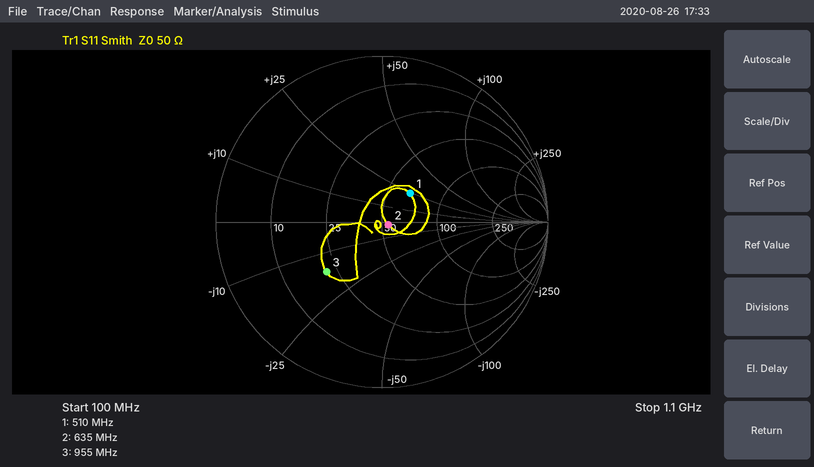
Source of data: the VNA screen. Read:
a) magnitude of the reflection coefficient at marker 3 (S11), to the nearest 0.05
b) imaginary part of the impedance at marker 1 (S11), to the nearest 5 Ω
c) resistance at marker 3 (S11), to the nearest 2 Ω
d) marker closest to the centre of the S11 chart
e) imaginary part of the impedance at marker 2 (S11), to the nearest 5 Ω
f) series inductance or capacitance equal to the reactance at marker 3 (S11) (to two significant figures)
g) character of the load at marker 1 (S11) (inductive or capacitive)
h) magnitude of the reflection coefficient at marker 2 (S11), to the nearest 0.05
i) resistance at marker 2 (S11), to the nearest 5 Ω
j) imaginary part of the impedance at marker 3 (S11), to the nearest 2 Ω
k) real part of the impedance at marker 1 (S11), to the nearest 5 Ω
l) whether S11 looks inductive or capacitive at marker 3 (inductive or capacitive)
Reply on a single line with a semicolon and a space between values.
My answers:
0.45; +25 Ω; 22 Ω; marker 2; 0 Ω; 10 pF; inductive; 0.05; 55 Ω; -16 Ω; 65 Ω; capacitive
